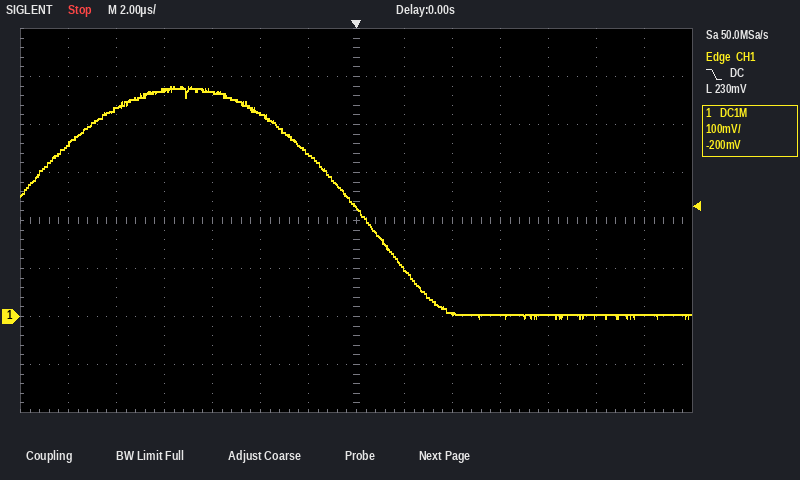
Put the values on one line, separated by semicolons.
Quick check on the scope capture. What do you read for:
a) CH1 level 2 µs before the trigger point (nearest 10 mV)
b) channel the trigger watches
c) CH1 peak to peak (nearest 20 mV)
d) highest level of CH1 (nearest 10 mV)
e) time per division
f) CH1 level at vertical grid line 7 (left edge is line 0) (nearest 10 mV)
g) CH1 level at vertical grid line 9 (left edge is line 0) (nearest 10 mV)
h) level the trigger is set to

340 mV; CH1; 480 mV; 480 mV; 2 µs; 230 mV; 10 mV; 230 mV
